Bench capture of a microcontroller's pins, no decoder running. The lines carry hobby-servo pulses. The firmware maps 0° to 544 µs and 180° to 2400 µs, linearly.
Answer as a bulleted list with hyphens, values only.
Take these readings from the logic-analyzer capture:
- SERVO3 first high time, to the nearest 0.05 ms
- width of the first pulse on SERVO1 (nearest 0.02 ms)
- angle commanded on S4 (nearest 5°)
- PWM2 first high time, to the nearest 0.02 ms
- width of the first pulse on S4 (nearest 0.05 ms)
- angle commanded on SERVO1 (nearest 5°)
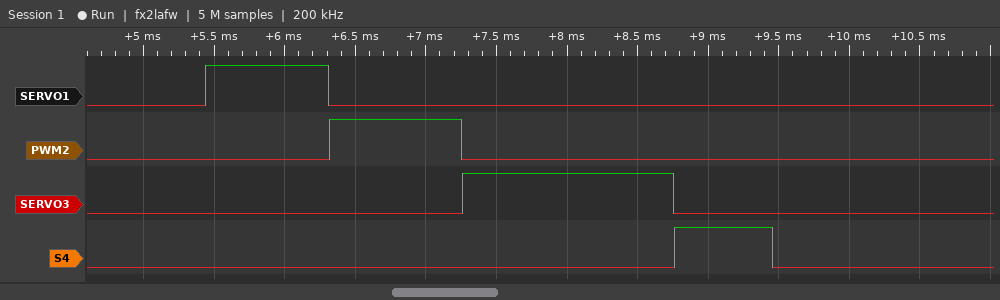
- 1.50 ms
- 0.86 ms
- 15°
- 0.94 ms
- 0.70 ms
- 30°
